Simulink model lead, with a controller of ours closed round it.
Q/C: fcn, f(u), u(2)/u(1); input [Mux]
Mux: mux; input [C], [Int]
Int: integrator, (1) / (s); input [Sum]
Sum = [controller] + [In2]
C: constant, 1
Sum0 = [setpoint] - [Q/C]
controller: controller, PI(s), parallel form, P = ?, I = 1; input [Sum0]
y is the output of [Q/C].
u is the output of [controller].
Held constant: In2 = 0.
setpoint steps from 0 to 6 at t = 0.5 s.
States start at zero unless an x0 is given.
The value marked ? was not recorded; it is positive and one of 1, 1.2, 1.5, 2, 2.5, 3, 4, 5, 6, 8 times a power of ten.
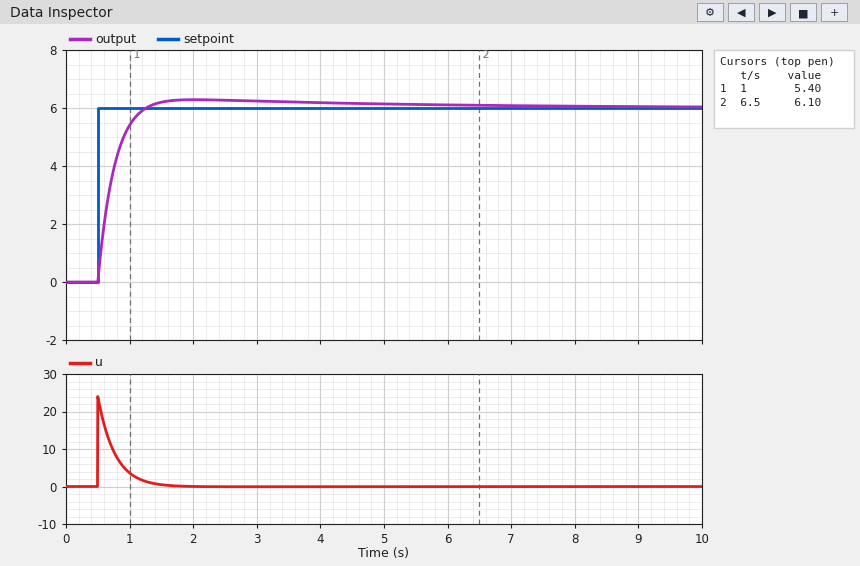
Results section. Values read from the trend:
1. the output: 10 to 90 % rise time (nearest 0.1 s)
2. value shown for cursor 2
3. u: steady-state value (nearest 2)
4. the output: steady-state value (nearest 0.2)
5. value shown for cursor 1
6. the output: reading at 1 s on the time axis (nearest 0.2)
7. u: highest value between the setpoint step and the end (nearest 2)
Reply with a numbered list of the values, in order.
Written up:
1. 0.5 s
2. 6.10
3. 0
4. 6.0
5. 5.40
6. 5.4
7. 24
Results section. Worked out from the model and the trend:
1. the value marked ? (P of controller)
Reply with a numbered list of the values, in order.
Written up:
1. 4
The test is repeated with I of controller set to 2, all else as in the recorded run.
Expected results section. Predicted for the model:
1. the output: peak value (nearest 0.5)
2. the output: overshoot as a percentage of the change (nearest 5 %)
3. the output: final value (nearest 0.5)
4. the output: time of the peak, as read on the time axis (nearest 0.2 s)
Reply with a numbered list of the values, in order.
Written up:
1. 6.5
2. 10 %
3. 6.0
4. 1.8 s
